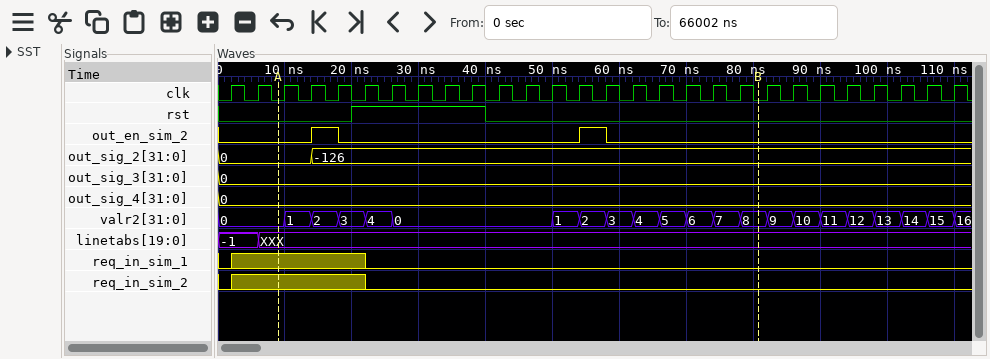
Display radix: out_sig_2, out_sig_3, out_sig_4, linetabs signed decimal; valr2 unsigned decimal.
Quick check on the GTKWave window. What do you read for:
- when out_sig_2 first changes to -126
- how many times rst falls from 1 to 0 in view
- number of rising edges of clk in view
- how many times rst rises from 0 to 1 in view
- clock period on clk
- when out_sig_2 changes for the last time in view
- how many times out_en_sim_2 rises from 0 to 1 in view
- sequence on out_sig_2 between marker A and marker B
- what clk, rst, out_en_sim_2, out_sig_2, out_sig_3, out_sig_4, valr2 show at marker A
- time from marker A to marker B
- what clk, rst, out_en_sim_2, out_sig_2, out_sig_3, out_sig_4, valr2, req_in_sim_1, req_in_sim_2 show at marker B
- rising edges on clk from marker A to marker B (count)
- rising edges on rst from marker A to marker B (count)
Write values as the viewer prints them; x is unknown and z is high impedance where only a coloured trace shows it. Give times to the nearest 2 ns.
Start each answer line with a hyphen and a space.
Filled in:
- 14 ns
- 1
- 28
- 1
- 4 ns
- 14 ns
- 2
- 0, -126
- clk=0, rst=0, out_en_sim_2=0, out_sig_2=0, out_sig_3=0, out_sig_4=0, valr2=0
- 72 ns
- clk=0, rst=0, out_en_sim_2=0, out_sig_2=-126, out_sig_3=0, out_sig_4=0, valr2=8, req_in_sim_1=0, req_in_sim_2=0
- 18
- 1
